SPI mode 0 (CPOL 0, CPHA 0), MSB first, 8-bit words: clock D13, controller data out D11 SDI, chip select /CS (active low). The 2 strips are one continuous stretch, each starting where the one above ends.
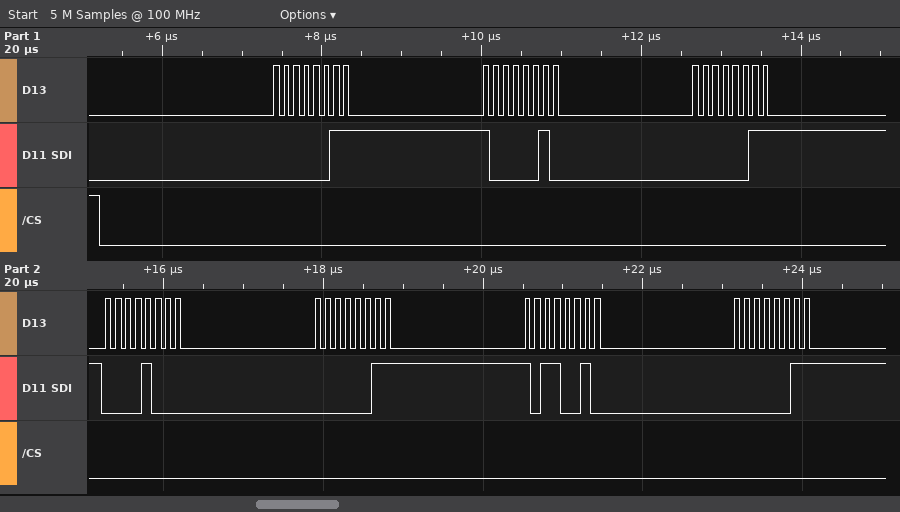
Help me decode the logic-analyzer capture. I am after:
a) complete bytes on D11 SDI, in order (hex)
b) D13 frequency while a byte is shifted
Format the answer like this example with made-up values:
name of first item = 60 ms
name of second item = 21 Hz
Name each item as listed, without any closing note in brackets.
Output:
complete bytes on D11 SDI, in order = 03 82 03 08 03 B2 03
D13 frequency while a byte is shifted = 8 MHz
